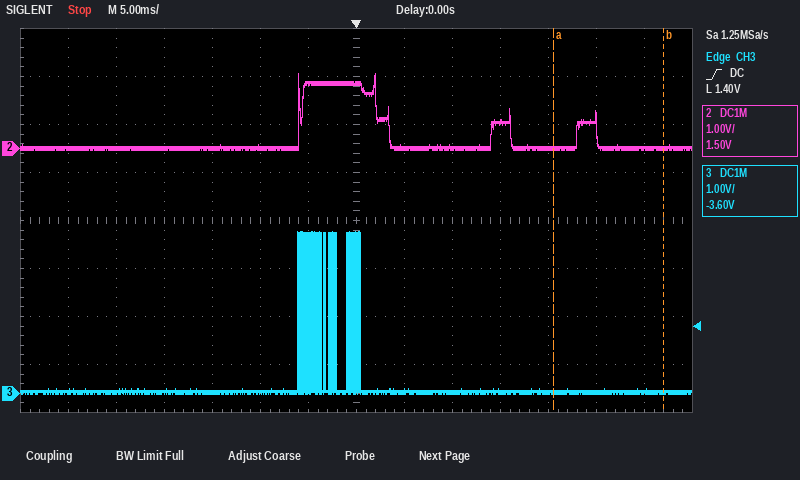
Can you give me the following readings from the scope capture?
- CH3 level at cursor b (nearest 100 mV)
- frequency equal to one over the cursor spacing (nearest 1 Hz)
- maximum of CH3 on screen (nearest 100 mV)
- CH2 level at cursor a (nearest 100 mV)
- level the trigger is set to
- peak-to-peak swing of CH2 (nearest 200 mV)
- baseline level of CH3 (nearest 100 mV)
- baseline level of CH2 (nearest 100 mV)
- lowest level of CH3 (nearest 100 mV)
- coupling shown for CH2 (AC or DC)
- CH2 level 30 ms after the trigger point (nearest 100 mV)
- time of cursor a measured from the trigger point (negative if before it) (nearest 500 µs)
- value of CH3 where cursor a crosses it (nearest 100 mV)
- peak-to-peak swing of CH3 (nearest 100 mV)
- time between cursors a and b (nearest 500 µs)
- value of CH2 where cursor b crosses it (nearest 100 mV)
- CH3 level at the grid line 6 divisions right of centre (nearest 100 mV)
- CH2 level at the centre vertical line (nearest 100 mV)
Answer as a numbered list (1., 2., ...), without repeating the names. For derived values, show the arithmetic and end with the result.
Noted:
1. 0.0 V
2. 1 / 11.5 ms ≈ 87 Hz
3. 3.4 V
4. 0.0 V
5. 1.40 V
6. 1.6 V
7. 0.0 V
8. 0.0 V
9. 0.0 V
10. DC
11. 0.0 V
12. +20.5 ms
13. 0.0 V
14. 3.4 V − (0.0 V) = 3.4 V
15. 11.5 ms
16. 0.0 V
17. 0.0 V
18. 1.4 V
